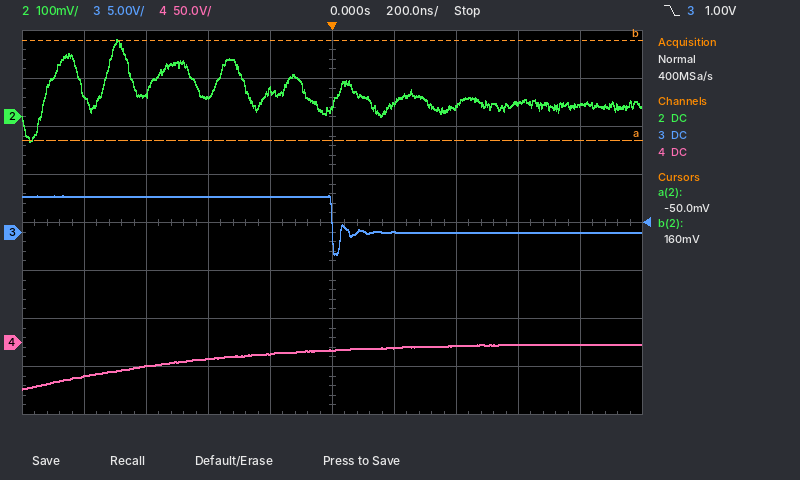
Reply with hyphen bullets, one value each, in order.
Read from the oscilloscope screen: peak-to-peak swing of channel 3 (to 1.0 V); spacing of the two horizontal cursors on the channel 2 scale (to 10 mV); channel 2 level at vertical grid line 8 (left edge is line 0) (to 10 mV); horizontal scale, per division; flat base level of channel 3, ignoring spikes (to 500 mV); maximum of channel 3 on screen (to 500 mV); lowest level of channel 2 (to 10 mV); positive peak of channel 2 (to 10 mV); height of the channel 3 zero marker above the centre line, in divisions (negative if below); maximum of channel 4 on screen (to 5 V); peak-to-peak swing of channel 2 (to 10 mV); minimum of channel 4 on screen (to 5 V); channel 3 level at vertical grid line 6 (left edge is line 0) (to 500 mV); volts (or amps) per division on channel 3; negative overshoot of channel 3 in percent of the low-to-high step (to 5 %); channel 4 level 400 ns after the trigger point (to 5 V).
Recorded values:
- 6.0 V
- 210 mV
- 30 mV
- 200 ns
- 0.0 V
- 4.0 V
- -50 mV
- 160 mV
- -0.2 div
- 0 V
- 210 mV
- -50 V
- 0.0 V
- 5 V
- 60 %
- -5 V
